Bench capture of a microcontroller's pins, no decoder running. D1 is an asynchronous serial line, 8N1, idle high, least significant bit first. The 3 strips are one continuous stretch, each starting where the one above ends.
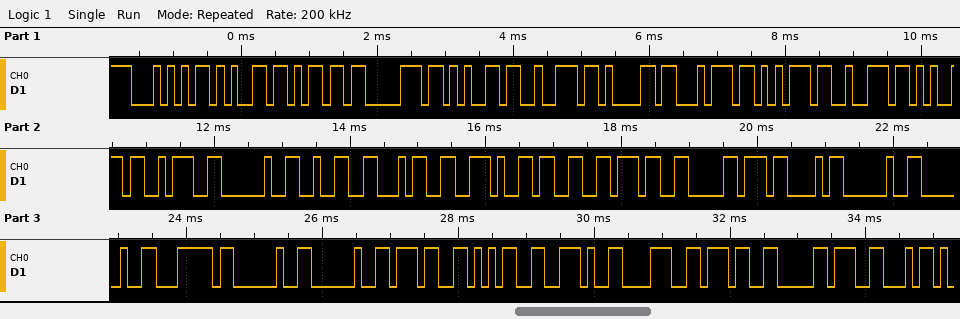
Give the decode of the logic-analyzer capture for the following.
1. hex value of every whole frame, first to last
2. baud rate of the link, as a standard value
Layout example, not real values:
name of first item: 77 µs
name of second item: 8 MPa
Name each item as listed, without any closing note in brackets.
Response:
hex value of every whole frame, first to last: 54 65 6D 70 65 72 61 74 75 72 65 3A 20 32 34 2E 33 37 B0 43 20 20 7C 20 20 37 35 2E 38 37 B0 46
baud rate of the link, as a standard value: 9600 baud
